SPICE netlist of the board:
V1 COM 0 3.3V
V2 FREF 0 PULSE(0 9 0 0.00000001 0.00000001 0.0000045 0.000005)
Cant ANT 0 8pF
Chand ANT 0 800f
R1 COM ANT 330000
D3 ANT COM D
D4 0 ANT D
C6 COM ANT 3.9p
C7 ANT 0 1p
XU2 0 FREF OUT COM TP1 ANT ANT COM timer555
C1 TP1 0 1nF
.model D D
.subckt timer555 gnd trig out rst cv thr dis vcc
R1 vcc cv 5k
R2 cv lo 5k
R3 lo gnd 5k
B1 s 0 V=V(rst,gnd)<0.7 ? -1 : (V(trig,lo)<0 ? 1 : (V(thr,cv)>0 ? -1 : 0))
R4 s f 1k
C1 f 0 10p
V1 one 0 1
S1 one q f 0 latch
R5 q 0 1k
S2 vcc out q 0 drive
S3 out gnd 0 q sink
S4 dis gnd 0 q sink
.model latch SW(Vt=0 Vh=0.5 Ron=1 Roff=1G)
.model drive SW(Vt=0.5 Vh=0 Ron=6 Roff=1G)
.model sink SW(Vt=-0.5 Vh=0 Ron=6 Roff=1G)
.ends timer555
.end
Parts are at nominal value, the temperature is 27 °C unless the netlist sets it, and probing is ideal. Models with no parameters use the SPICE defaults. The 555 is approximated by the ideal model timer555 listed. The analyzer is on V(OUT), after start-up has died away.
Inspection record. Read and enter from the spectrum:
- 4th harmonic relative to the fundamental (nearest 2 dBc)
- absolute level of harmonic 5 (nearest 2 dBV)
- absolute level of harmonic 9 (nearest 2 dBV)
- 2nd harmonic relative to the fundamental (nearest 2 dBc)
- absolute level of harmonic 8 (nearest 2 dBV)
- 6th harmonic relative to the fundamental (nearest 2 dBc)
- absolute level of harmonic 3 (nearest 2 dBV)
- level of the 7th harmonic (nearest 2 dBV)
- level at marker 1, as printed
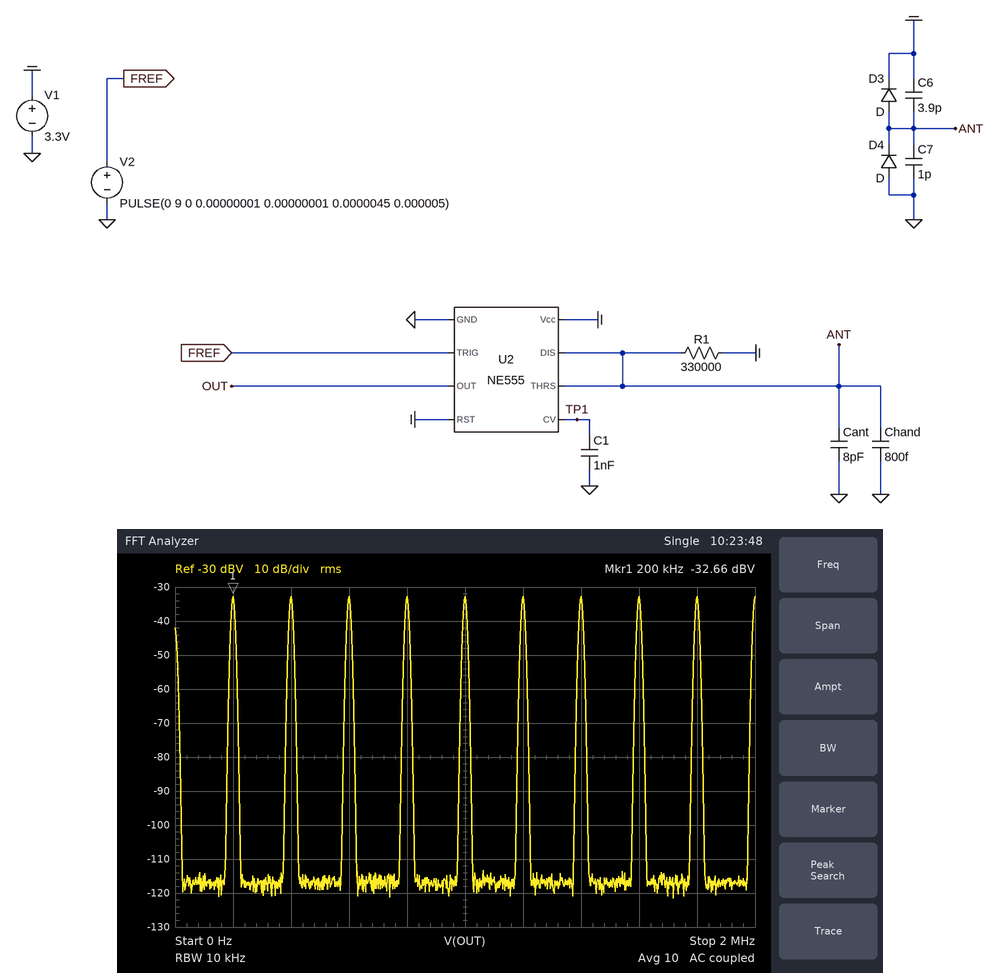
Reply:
0 dBc
-32 dBV
-32 dBV
0 dBc
-32 dBV
0 dBc
-32 dBV
-32 dBV
-32.66 dBV
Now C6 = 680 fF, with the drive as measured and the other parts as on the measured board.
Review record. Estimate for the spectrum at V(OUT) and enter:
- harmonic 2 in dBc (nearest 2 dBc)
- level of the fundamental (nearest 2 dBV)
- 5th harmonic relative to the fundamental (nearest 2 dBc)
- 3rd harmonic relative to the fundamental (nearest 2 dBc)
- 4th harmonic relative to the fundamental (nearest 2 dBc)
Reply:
-2 dBc
0 dBV
-16 dBc
-8 dBc
-26 dBc
